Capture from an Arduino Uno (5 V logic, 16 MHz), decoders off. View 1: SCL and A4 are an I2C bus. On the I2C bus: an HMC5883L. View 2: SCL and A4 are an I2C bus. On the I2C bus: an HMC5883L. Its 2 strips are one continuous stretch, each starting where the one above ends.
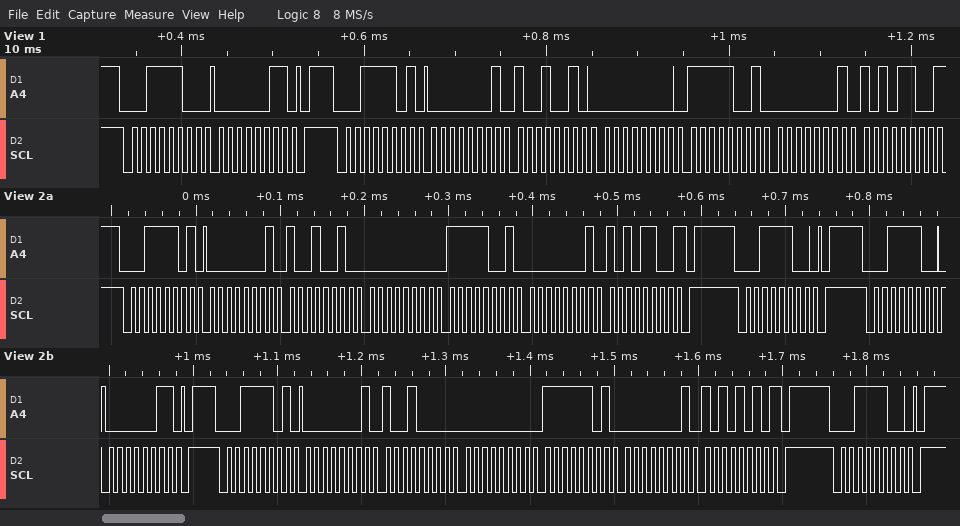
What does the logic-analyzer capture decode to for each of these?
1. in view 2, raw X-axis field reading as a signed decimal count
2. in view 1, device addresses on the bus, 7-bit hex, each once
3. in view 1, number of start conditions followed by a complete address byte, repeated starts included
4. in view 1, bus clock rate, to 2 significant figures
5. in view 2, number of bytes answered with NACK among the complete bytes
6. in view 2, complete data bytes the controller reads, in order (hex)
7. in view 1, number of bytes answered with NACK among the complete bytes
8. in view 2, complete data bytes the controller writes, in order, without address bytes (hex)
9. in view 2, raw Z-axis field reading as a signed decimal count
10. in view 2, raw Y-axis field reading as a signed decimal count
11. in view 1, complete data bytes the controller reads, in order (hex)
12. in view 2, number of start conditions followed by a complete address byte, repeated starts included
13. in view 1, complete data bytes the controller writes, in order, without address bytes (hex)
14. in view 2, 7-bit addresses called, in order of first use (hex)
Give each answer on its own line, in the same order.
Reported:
400
0x1E
2
100 kHz
2
01 92 00 F9 01 AC 01 90 00 FD 01 AA
1
03
253
426
01 92 00 F9 01 AC
5
03
0x1E
